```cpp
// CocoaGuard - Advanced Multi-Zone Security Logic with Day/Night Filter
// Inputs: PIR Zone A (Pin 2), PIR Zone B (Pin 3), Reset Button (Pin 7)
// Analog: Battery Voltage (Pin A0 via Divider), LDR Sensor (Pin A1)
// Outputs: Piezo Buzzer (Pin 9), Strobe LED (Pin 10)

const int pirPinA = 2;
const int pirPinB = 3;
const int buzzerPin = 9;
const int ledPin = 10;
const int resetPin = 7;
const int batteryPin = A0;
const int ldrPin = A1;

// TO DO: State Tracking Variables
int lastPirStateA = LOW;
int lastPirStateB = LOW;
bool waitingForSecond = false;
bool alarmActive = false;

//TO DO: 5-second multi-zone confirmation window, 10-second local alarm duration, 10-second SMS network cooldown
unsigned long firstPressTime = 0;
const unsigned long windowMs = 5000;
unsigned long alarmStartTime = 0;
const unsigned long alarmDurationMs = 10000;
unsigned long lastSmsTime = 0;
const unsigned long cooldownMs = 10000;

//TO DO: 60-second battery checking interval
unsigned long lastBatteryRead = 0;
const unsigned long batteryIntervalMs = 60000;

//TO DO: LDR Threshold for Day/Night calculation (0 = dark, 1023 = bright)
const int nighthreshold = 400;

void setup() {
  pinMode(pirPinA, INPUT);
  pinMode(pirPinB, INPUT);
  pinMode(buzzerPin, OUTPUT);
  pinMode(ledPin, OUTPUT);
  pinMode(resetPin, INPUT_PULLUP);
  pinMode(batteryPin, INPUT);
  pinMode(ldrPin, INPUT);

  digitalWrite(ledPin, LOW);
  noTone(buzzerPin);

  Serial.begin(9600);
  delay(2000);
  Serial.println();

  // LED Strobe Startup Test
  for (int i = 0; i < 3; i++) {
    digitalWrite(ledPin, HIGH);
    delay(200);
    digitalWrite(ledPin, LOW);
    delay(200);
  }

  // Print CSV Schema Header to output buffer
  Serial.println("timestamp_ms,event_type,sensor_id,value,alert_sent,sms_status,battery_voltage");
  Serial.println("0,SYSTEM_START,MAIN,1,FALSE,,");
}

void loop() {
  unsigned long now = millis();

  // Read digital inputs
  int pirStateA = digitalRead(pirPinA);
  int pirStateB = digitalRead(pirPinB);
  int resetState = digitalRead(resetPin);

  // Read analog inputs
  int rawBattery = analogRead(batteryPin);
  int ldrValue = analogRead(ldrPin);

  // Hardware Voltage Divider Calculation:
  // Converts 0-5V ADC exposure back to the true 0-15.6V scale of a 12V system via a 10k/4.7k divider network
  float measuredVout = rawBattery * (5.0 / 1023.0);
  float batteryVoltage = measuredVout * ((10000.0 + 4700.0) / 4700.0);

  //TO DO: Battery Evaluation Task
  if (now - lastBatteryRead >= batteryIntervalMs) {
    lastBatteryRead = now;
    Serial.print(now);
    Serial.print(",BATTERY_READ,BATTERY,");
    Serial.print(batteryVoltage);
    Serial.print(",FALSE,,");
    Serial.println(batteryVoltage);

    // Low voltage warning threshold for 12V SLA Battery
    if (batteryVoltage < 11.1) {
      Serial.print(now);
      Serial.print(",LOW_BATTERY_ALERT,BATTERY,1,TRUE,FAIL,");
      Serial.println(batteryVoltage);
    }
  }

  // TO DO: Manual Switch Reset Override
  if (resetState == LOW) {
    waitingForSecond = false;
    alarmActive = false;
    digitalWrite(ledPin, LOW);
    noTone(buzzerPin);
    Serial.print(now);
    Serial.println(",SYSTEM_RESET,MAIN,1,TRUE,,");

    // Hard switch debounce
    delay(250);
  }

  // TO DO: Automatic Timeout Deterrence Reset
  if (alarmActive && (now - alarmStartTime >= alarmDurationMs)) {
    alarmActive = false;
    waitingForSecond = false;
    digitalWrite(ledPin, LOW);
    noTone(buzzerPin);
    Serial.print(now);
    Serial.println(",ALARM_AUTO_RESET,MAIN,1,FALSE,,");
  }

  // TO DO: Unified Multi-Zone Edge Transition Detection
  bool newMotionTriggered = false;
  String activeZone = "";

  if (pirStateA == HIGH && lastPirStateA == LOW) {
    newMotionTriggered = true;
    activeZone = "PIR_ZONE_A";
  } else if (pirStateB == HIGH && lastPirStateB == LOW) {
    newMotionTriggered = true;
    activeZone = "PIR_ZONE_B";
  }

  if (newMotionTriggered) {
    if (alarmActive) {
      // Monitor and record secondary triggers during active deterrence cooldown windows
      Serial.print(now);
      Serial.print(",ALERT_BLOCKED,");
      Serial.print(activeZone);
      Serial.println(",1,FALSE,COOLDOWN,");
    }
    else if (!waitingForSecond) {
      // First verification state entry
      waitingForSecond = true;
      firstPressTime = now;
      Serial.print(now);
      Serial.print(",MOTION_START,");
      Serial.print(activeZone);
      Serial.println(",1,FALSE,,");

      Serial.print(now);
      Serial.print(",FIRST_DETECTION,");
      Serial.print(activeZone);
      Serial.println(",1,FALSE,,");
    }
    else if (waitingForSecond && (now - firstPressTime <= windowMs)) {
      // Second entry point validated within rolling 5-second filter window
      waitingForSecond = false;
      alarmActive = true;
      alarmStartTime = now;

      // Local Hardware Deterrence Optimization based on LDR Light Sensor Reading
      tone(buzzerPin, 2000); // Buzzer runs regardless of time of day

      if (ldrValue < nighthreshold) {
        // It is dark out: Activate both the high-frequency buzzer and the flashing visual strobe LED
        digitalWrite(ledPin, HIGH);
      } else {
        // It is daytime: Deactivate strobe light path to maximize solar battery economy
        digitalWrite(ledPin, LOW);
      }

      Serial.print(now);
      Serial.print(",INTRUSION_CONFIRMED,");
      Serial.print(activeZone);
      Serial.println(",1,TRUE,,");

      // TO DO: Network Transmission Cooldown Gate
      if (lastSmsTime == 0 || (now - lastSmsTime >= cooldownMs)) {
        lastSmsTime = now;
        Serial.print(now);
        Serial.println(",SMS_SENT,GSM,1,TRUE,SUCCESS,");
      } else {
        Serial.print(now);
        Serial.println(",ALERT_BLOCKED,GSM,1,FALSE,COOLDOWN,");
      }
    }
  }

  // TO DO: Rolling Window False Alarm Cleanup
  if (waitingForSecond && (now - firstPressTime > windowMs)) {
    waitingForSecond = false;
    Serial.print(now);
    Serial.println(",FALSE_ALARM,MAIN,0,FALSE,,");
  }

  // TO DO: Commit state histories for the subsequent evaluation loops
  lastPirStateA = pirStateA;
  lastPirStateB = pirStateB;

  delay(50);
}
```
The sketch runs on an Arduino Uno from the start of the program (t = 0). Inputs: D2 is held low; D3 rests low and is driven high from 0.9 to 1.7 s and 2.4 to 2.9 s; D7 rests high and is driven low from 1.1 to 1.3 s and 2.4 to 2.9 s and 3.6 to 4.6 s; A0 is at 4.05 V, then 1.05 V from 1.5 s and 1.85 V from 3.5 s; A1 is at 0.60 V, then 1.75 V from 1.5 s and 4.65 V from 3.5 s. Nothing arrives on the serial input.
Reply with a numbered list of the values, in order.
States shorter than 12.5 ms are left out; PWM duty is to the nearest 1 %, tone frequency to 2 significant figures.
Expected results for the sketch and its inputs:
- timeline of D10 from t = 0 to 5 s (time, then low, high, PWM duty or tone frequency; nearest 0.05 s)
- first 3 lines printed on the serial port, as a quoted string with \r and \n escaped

1. 0 s low; 2 s high; 2.2 s low; 2.4 s high; 2.6 s low; 2.8 s high; 3 s low
2. "\r\ntimestamp_ms,event_type,sensor_id,value,alert_sent,sms_status,battery_voltage\r\n0,SYSTEM_START,MAIN,1,FALSE,,\r\n"
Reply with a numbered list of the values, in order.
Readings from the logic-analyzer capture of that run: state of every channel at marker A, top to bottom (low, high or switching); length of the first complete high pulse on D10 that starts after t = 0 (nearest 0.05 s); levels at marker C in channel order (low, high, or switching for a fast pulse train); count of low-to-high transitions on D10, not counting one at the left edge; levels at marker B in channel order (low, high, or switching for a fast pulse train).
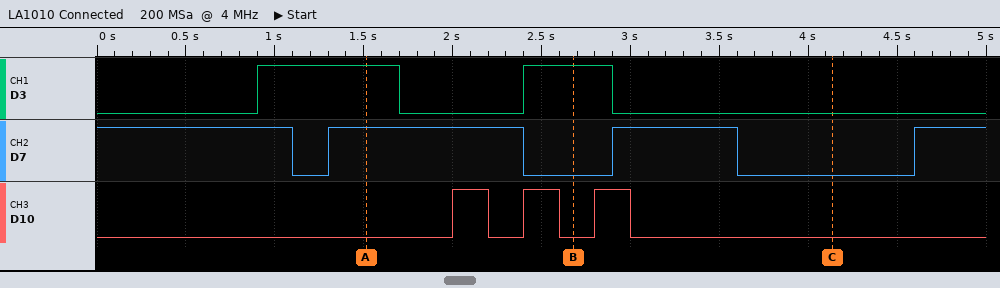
1. D3 high, D7 high, D10 low
2. 0.20 s
3. D3 low, D7 low, D10 low
4. 3
5. D3 high, D7 low, D10 low
